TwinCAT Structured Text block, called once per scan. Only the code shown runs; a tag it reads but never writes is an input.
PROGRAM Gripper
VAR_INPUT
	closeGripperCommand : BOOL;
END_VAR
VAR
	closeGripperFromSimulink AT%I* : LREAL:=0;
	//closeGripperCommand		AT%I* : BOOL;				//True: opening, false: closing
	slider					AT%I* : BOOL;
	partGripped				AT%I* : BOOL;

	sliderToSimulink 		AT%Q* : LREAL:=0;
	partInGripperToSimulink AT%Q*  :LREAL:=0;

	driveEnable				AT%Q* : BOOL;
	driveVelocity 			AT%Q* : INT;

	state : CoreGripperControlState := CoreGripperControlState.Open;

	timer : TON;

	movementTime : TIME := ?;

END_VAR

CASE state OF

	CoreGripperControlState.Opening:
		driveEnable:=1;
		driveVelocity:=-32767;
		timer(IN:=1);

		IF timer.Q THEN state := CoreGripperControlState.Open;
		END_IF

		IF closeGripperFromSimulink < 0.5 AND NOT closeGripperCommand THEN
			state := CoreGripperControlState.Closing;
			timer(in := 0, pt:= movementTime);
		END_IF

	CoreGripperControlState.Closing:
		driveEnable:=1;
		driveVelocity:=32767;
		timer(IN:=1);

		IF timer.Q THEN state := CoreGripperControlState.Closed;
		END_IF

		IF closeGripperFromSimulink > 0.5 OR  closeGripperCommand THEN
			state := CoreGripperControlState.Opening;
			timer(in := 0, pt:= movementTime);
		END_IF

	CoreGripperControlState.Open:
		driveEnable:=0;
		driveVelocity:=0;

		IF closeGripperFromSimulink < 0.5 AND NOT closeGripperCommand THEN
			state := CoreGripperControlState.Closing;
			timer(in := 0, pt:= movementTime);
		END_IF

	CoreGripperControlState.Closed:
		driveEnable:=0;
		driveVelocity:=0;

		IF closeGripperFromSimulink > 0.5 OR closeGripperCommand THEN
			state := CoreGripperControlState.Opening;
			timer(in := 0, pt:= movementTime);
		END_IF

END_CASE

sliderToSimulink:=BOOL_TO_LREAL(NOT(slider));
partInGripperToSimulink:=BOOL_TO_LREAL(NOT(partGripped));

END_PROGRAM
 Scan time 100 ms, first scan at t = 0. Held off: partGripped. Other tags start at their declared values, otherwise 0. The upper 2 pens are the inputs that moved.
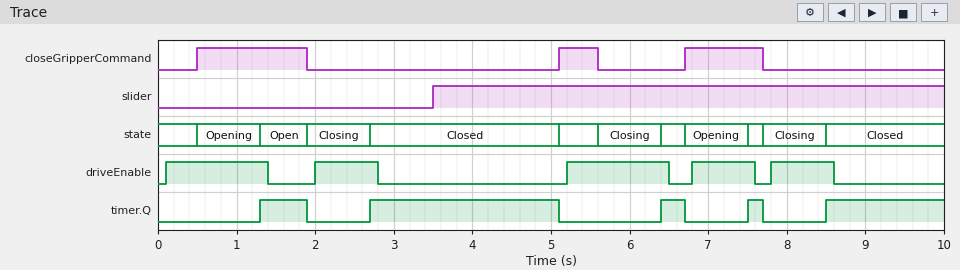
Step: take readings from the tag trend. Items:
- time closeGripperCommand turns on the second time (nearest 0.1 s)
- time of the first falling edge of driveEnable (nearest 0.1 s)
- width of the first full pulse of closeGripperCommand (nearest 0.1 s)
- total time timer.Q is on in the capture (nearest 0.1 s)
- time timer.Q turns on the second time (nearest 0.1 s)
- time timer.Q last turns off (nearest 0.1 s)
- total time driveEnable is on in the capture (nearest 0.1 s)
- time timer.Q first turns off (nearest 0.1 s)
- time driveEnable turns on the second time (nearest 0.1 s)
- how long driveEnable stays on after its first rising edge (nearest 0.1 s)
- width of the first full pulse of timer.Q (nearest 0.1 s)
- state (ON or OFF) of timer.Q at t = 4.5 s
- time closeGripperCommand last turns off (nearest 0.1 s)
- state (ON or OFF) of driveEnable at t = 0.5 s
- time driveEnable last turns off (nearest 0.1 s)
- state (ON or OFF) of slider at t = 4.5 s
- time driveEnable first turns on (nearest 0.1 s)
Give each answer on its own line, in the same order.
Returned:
5.1 s
1.4 s
1.4 s
5.0 s
2.7 s
7.7 s
5.0 s
1.9 s
2.0 s
1.3 s
0.6 s
ON
7.7 s
ON
8.6 s
ON
0.1 s
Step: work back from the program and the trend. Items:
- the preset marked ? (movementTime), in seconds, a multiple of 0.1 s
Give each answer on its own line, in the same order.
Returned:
0.7 s
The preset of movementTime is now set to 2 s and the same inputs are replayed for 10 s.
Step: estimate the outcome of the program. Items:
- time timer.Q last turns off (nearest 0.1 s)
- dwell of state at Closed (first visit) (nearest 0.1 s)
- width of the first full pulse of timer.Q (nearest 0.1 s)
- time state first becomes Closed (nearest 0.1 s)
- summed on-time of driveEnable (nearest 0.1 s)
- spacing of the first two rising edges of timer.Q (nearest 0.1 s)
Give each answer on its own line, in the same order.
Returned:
5.1 s
1.1 s
1.1 s
4.0 s
8.7 s
5.8 s
